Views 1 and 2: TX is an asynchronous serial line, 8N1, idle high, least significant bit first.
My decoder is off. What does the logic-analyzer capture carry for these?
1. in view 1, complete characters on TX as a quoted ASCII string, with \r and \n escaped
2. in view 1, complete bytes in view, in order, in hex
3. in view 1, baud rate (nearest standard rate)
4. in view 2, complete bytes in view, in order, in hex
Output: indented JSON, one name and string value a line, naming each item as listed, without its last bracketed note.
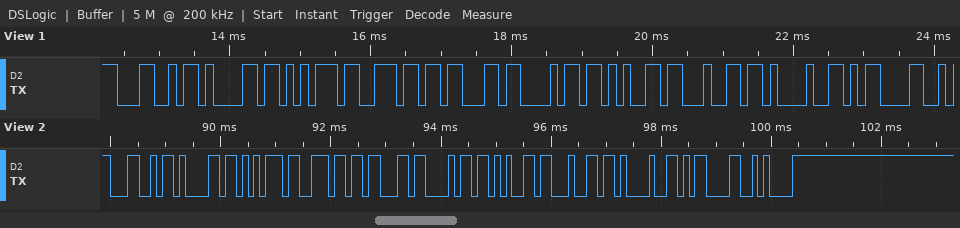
{
  "in view 1, complete characters on TX as a quoted ASCII string, with \\r and \\n escaped": "\"Launched!\\r\"",
  "in view 1, complete bytes in view, in order, in hex": "0x4C 0x61 0x75 0x6E 0x63 0x68 0x65 0x64 0x21 0x0D",
  "in view 1, baud rate": "9600 baud",
  "in view 2, complete bytes in view, in order, in hex": "4C 61 75 6E 63 68 65 64 21 0D 0A"
}
